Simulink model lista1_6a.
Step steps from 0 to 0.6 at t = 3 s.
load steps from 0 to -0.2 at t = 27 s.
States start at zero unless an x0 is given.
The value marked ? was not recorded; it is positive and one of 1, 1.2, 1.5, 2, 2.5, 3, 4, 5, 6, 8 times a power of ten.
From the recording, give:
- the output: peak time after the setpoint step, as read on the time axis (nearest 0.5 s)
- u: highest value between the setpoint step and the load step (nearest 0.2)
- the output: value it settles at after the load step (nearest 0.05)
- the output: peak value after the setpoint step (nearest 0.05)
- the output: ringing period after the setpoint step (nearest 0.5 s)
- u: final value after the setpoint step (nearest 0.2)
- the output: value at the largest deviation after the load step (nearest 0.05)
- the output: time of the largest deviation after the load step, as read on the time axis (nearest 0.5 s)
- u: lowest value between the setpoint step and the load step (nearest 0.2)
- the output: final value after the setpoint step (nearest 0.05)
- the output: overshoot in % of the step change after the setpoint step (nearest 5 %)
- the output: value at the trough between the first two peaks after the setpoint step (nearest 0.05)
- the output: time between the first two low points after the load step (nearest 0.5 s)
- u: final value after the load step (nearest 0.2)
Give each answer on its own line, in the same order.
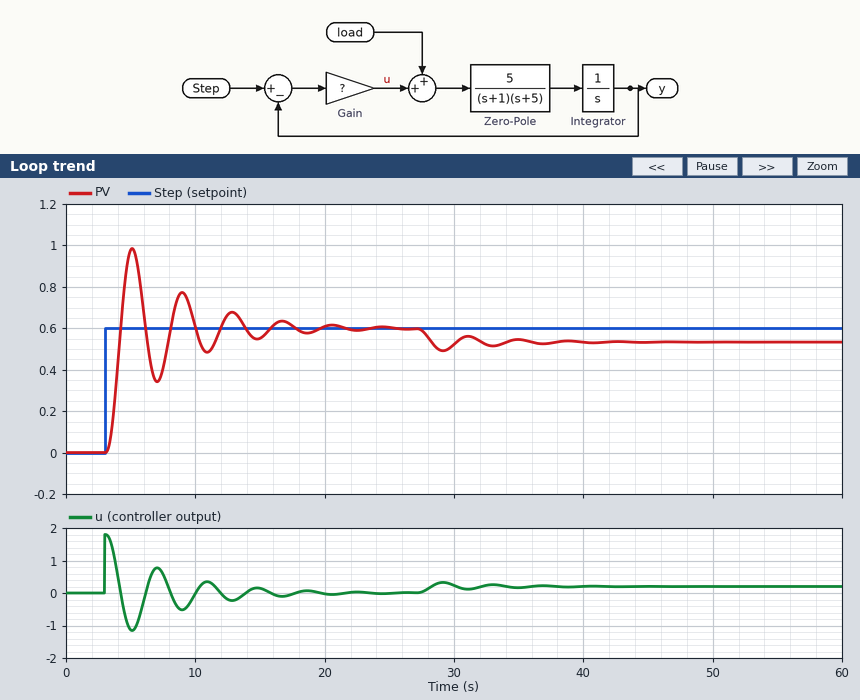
5.0 s
1.8
0.55
1.00
4.0 s
0.0
0.50
29.0 s
-1.2
0.60
65 %
0.35
4.0 s
0.2
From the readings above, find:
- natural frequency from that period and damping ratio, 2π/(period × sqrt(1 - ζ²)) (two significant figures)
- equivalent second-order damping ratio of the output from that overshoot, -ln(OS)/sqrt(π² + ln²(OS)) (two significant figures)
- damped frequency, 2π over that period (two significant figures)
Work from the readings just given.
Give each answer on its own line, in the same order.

1.6 rad/s
0.14
1.6 rad/s
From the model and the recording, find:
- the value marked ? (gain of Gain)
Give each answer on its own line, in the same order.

3
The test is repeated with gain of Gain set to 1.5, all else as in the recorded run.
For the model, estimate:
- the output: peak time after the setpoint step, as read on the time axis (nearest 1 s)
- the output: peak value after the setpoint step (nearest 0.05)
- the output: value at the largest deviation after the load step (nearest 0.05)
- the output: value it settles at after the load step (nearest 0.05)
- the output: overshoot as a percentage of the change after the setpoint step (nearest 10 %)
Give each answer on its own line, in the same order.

6 s
0.85
0.40
0.45
40 %
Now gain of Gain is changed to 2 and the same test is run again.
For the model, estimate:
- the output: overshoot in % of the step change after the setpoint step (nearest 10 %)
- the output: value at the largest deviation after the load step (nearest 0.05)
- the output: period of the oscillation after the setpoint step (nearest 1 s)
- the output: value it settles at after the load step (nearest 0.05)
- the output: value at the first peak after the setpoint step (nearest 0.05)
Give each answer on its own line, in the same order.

50 %
0.45
5 s
0.50
0.90
